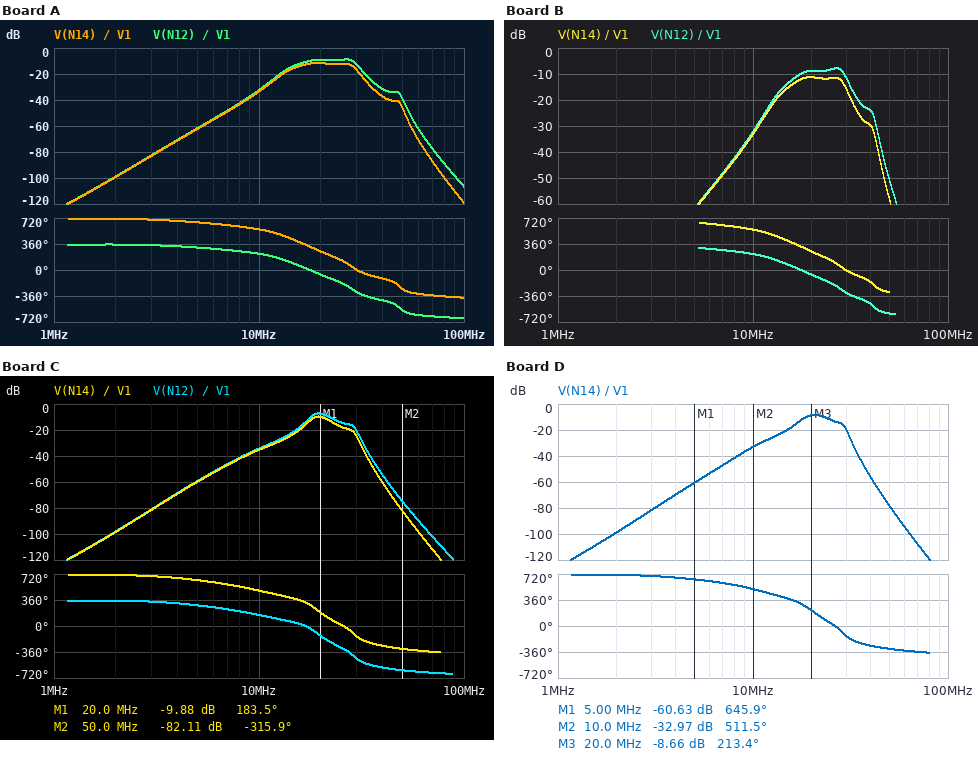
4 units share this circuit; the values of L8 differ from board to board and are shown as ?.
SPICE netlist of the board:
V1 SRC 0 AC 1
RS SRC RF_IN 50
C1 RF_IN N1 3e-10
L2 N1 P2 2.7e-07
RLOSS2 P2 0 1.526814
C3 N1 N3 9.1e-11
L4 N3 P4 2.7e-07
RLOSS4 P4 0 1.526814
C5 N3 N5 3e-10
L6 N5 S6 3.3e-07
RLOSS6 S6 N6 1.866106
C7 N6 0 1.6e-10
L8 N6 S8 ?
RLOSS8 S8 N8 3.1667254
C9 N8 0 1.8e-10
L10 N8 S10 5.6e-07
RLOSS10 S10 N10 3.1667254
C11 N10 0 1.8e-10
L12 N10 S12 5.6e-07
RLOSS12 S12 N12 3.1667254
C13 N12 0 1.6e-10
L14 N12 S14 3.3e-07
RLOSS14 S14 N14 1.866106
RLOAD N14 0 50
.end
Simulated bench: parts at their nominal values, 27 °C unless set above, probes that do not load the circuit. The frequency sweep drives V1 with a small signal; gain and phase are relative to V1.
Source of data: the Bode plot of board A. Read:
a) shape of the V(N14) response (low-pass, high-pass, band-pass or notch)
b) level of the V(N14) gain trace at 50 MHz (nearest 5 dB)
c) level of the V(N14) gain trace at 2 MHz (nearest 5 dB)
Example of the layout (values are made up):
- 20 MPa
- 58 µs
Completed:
- band-pass
- -45 dB
- -100 dB
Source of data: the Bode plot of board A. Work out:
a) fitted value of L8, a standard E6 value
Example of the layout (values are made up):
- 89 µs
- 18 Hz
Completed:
- 150 nH
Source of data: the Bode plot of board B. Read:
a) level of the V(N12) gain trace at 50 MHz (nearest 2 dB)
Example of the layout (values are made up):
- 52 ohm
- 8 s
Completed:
- -50 dB
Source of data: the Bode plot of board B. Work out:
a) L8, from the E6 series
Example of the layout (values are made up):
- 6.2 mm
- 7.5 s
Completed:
- 220 nH
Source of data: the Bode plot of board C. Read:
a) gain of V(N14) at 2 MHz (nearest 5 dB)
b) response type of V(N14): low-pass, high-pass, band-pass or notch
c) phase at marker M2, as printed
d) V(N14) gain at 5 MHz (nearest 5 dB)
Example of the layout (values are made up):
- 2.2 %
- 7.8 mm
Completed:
- -100 dB
- band-pass
- -315.9 deg
- -60 dB
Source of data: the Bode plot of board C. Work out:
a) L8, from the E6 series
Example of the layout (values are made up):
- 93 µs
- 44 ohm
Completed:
- 1.5 µH
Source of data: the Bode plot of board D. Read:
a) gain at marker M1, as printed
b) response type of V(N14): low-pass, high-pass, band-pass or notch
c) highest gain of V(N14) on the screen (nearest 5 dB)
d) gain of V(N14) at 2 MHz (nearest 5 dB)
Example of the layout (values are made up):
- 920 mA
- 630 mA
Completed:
- -60.63 dB
- band-pass
- -10 dB
- -100 dB
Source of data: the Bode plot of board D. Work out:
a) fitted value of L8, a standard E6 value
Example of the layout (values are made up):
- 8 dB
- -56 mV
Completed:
- 1 µH
